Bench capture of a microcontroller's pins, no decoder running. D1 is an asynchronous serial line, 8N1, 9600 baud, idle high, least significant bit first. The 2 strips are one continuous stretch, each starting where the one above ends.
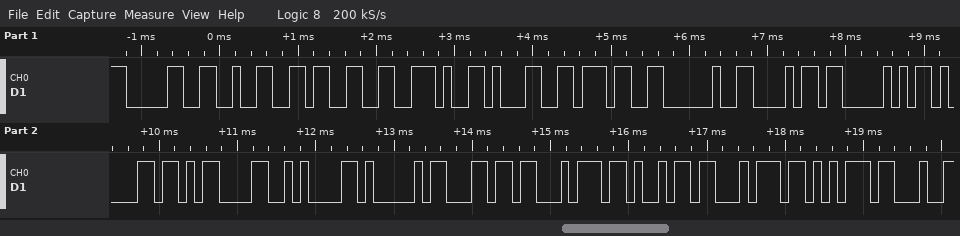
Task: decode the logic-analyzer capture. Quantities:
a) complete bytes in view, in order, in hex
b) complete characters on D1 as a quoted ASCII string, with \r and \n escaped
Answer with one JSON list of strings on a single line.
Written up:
["30 32 33 2E 31 37 20 68 50 61 0D 0A 41 6C 74 69 74 75", "\"023.17 hPa\\r\\nAltitu\""]
